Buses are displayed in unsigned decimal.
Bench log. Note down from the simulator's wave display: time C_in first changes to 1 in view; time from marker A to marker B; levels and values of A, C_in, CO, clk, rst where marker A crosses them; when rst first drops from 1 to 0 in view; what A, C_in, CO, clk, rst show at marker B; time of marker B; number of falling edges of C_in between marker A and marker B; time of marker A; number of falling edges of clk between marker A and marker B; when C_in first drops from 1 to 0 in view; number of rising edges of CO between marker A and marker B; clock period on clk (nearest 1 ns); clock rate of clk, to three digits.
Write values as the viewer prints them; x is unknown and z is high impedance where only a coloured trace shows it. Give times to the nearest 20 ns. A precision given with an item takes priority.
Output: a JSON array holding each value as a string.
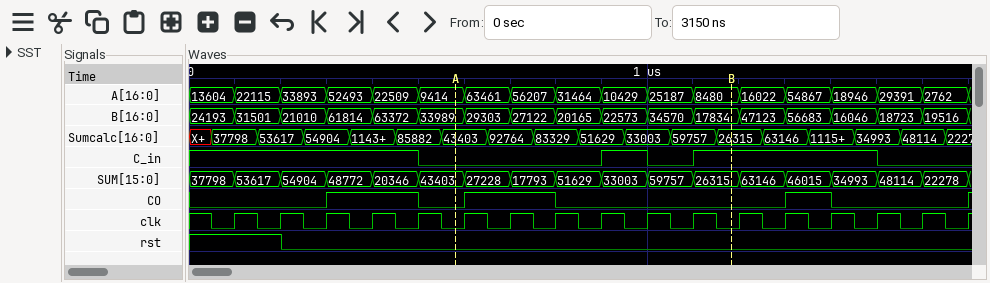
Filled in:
["900 ns", "600 ns", "A=9414, C_in=0, CO=0, clk=0, rst=0", "200 ns", "A=8480, C_in=1, CO=0, clk=0, rst=0", "1180 ns", "1", "580 ns", "6", "500 ns", "1", "100 ns", "10.0 MHz"]
